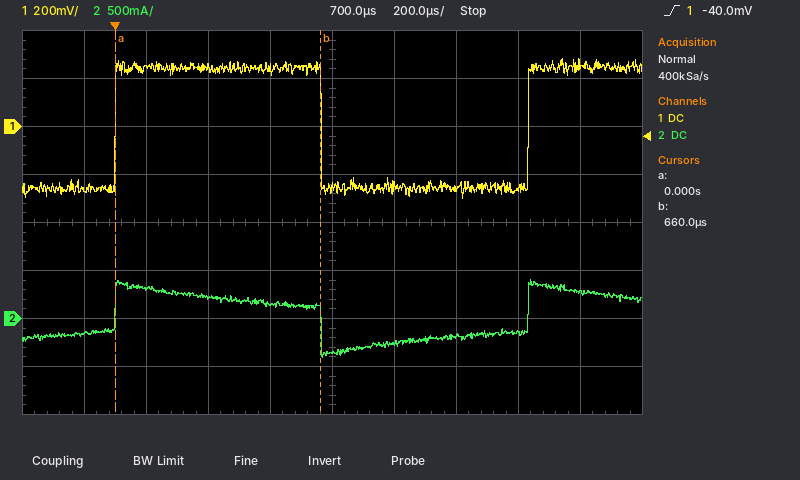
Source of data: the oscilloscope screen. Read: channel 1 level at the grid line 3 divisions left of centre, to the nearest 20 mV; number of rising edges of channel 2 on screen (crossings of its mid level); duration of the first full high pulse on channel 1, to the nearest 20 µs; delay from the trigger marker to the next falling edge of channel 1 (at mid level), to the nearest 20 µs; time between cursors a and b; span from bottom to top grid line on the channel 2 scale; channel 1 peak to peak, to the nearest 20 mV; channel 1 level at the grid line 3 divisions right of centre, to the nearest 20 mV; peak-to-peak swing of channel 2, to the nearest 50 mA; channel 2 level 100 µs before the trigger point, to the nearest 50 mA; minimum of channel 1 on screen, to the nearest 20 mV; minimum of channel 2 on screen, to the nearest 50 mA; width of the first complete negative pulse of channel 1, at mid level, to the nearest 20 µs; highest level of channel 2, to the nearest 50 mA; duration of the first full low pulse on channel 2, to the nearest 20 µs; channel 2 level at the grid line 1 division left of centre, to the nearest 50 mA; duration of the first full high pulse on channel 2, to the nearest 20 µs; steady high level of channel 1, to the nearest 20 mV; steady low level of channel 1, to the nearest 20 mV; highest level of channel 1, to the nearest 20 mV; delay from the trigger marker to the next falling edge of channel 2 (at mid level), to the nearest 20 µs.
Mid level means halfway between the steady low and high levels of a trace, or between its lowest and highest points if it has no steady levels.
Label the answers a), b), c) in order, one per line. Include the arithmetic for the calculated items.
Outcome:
a) 240 mV
b) 2
c) 660 µs
d) 660 µs
e) 660 µs − (0 s) = 660 µs
f) 4 A
g) 280 mV − (-300 mV) = 580 mV
h) -260 mV
i) 400 mA − (-400 mA) = 800 mA
j) -150 mA
k) -300 mV
l) -400 mA
m) 660 µs
n) 400 mA
o) 660 µs
p) 150 mA
q) 660 µs
r) 240 mV
s) -260 mV
t) 280 mV
u) 660 µs
